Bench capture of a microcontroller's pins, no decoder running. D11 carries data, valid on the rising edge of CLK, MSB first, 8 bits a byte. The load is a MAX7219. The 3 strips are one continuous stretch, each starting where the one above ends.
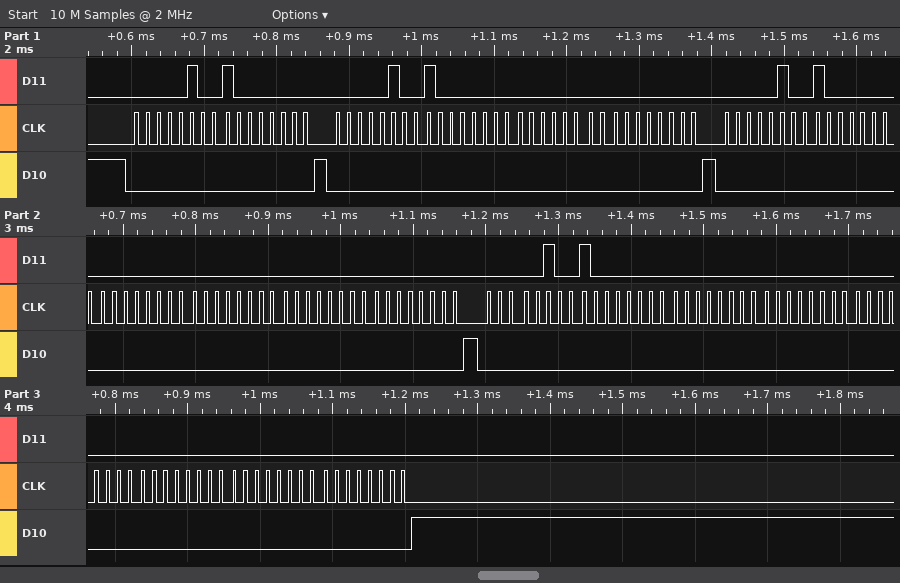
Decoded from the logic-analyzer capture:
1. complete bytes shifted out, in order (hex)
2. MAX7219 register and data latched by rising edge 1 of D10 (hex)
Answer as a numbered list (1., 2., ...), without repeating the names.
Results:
1. 04 80 04 80 00 00 04 80 00 00 00 00 04 80 00 00 00 00 00 00
2. register 0x4, data 0x80
